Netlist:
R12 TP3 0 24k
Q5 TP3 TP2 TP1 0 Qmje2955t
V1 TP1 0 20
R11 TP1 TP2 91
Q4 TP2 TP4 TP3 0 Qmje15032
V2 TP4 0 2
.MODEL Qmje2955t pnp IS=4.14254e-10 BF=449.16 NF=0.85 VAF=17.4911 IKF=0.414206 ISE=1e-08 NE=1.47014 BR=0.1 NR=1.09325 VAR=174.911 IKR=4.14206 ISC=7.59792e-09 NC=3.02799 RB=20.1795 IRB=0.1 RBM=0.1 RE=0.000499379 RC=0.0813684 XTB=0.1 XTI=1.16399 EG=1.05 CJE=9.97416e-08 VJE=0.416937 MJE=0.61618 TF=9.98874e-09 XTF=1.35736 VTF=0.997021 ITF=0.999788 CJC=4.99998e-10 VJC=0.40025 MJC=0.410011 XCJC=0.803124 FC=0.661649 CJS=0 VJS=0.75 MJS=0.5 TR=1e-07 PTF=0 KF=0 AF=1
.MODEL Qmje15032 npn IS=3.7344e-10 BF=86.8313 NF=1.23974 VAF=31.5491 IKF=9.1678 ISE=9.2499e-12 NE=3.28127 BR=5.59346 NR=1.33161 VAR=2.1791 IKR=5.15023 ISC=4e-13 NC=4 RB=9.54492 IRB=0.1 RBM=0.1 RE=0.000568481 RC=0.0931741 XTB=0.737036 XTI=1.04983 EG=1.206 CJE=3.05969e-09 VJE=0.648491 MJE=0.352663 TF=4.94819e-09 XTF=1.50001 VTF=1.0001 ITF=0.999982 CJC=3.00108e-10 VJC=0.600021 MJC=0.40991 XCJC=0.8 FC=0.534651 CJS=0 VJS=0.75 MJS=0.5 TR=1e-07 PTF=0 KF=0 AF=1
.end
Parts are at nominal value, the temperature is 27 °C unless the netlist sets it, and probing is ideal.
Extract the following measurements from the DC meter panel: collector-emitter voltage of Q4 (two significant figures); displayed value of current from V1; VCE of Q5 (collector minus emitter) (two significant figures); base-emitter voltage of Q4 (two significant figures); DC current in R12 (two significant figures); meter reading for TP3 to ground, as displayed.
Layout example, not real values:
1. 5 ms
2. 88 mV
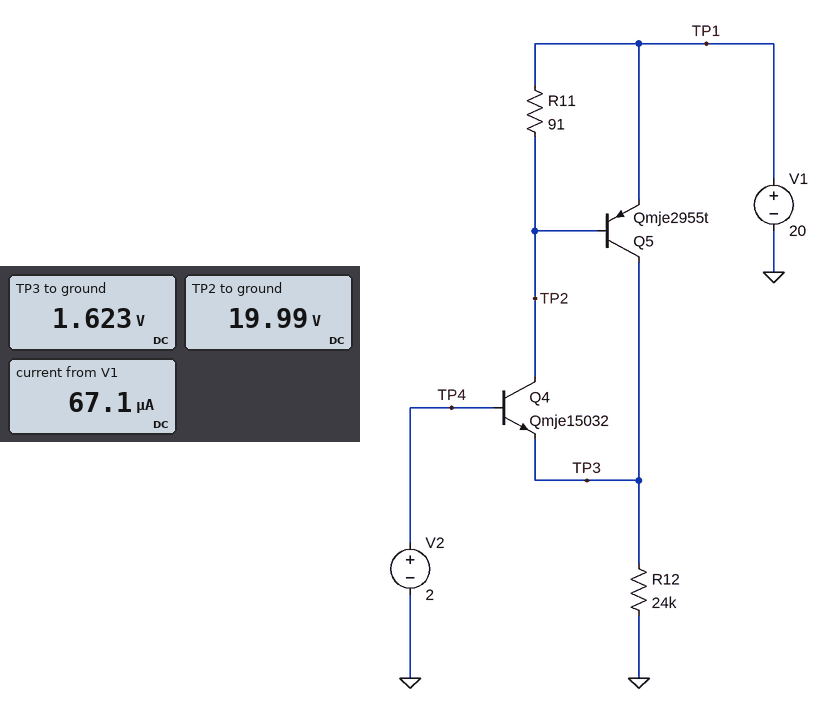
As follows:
1. 18 V
2. 67.1 µA
3. -18 V
4. 380 mV
5. 68 µA
6. 1.623 V
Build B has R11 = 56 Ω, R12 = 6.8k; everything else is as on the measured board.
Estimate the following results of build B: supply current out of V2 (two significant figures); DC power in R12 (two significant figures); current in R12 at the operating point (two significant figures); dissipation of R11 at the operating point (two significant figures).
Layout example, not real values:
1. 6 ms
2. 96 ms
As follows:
1. 1.9 µA
2. 370 µW
3. 230 µA
4. 3.0 µW
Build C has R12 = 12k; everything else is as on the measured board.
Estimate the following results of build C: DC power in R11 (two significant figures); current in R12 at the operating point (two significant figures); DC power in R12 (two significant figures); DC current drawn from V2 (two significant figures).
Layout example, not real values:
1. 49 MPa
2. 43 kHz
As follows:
1. 1.6 µW
2. 130 µA
3. 210 µW
4. 1.1 µA
